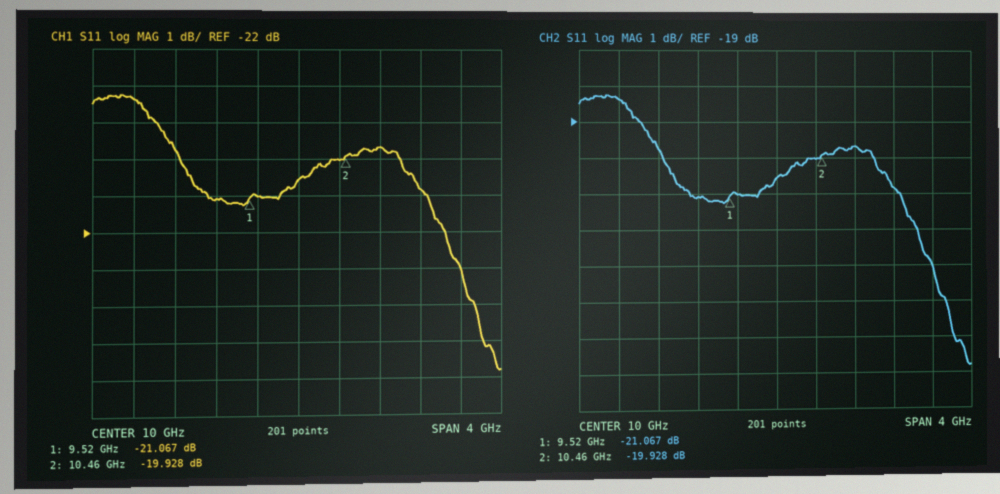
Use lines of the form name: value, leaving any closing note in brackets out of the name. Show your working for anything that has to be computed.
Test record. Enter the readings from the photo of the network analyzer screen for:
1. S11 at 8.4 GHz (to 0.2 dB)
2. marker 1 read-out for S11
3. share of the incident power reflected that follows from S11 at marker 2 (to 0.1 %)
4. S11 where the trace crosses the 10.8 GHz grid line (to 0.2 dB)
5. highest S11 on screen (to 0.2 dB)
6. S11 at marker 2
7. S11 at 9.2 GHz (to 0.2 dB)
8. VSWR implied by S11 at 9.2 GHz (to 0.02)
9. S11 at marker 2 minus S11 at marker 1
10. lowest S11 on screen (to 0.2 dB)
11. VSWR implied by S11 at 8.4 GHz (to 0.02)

S11 at 8.4 GHz: -18.4 dB
marker 1 read-out for S11: -21.067 dB
share of the incident power reflected that follows from S11 at marker 2: 10^(-19.928/10) ≈ 1.0 %
S11 where the trace crosses the 10.8 GHz grid line: -19.6 dB
highest S11 on screen: -18.2 dB
S11 at marker 2: -19.928 dB
S11 at 9.2 GHz: -21.0 dB
VSWR implied by S11 at 9.2 GHz: |Γ| = 10^(-21/20) = 0.0891; VSWR = (1 + 0.0891)/(1 − 0.0891) ≈ 1.20
S11 at marker 2 minus S11 at marker 1: -19.928 − (-21.067) = 1.139 dB
lowest S11 on screen: -25.8 dB
VSWR implied by S11 at 8.4 GHz: |Γ| = 10^(-18.4/20) = 0.1202; VSWR = (1 + 0.1202)/(1 − 0.1202) ≈ 1.27, so 1.28 to the nearest 0.02
